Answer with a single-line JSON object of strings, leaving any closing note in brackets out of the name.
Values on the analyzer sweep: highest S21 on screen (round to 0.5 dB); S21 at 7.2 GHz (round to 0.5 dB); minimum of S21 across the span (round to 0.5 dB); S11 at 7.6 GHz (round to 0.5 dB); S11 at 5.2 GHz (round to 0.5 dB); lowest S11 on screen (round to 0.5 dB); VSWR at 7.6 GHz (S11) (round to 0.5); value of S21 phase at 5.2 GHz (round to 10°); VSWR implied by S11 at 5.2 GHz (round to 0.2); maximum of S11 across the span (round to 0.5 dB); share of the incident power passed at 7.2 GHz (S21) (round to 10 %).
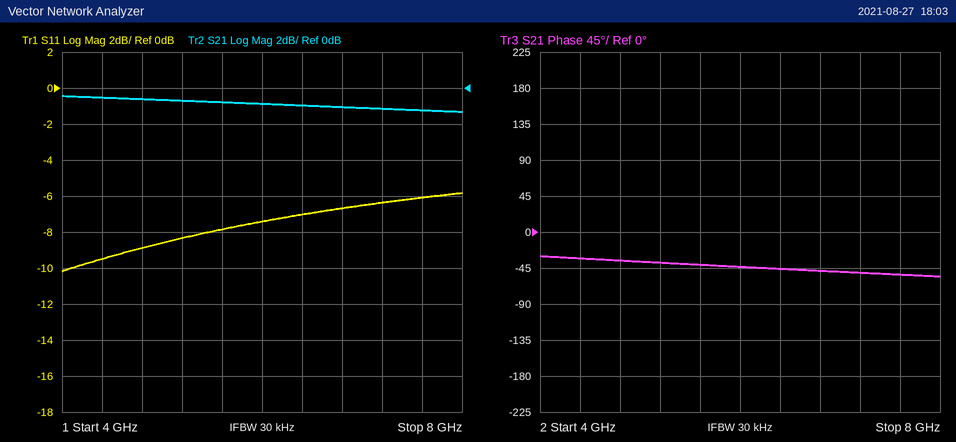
{"highest S21 on screen": "-0.5 dB", "S21 at 7.2 GHz": "-1.0 dB", "minimum of S21 across the span": "-1.5 dB", "S11 at 7.6 GHz": "-6.0 dB", "S11 at 5.2 GHz": "-8.5 dB", "lowest S11 on screen": "-10.0 dB", "VSWR at 7.6 GHz (S11)": "3.0", "value of S21 phase at 5.2 GHz": "-40°", "VSWR implied by S11 at 5.2 GHz": "2.2", "maximum of S11 across the span": "-6.0 dB", "share of the incident power passed at 7.2 GHz (S21)": "80 %"}
